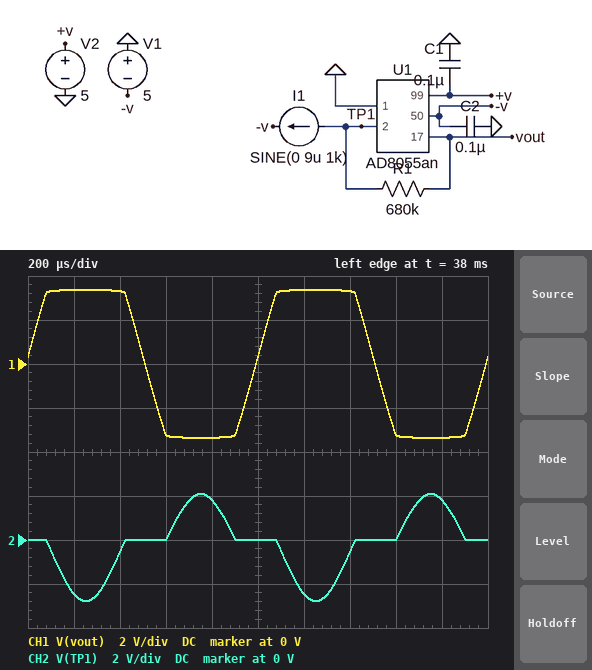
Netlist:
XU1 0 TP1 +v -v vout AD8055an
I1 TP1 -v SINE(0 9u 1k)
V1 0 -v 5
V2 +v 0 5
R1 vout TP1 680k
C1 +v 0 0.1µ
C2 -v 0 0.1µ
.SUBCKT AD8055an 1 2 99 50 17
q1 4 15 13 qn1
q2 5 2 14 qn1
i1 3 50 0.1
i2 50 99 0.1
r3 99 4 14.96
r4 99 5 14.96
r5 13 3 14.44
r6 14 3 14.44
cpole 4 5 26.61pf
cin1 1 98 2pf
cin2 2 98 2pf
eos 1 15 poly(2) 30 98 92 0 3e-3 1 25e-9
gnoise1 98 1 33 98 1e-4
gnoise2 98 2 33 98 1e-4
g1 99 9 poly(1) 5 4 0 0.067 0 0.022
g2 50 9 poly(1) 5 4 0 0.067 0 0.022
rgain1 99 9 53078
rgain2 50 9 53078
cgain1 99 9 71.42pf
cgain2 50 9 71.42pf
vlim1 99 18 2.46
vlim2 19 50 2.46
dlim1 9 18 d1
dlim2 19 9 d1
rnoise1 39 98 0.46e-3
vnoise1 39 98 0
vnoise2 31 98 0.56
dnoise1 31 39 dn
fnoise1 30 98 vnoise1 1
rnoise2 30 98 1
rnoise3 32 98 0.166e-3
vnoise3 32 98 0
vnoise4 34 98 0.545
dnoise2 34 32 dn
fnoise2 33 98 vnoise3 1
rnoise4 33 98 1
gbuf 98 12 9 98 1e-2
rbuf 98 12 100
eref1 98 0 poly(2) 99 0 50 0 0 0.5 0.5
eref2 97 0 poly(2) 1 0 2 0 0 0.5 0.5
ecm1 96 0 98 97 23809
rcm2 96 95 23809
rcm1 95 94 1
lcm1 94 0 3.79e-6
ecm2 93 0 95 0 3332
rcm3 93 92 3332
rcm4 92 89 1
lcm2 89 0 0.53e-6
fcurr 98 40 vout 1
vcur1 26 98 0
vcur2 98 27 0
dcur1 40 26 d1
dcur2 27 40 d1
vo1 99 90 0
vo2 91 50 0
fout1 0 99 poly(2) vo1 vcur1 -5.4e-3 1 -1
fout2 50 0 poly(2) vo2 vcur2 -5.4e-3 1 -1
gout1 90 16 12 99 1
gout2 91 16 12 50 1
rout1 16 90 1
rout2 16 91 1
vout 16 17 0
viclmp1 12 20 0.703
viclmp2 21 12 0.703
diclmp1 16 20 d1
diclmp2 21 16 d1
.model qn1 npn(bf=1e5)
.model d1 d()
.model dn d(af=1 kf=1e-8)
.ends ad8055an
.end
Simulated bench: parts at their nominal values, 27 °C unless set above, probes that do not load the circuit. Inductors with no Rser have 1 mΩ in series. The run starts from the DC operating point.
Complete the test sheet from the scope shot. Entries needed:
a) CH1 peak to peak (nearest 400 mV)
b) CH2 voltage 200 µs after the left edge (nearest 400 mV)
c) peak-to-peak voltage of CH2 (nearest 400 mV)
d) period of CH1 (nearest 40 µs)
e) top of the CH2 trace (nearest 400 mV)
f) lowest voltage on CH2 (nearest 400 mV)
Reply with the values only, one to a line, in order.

6.8 V
-2.4 V
4.8 V
1.00 ms
2.0 V
-2.8 V
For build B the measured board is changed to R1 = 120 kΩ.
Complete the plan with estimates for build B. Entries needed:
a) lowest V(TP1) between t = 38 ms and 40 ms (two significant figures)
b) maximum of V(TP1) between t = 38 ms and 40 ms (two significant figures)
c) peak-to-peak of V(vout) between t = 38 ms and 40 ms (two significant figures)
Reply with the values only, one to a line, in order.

-3.3 mV
-2.7 mV
2.2 V
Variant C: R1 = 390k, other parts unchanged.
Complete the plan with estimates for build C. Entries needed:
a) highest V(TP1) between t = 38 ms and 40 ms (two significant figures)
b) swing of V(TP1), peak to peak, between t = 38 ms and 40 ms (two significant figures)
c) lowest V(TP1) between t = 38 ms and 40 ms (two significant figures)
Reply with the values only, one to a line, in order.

58 mV
420 mV
-360 mV
